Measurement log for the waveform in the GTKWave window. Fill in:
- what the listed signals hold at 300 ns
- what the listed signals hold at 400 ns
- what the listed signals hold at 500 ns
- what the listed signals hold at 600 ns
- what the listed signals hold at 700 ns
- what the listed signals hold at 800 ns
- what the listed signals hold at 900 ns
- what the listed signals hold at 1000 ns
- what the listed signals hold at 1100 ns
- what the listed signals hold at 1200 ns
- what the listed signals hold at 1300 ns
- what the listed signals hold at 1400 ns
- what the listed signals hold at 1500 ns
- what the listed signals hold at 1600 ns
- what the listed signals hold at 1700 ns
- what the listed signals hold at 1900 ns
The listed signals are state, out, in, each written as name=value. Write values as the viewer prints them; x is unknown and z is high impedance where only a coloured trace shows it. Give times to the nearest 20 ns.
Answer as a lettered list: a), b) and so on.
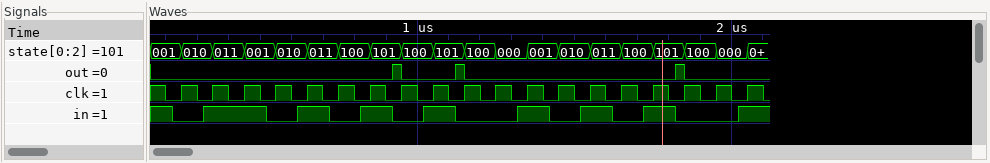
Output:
a) state=010, out=0, in=0
b) state=011, out=0, in=1
c) state=001, out=0, in=1
d) state=010, out=0, in=0
e) state=011, out=0, in=1
f) state=100, out=0, in=0
g) state=101, out=0, in=1
h) state=100, out=0, in=0
i) state=101, out=0, in=1
j) state=100, out=0, in=0
k) state=000, out=0, in=0
l) state=001, out=0, in=1
m) state=010, out=0, in=0
n) state=011, out=0, in=1
o) state=100, out=0, in=0
p) state=100, out=0, in=0
